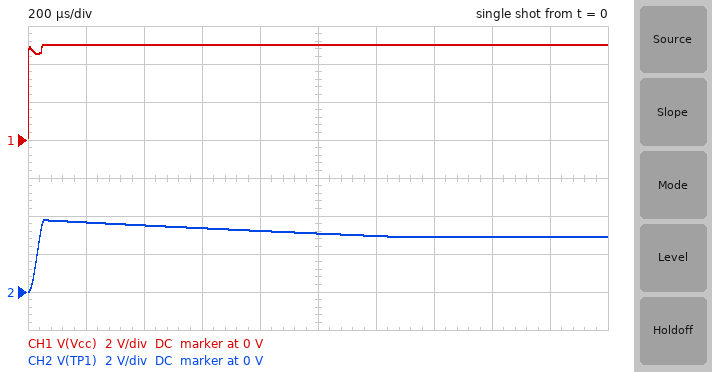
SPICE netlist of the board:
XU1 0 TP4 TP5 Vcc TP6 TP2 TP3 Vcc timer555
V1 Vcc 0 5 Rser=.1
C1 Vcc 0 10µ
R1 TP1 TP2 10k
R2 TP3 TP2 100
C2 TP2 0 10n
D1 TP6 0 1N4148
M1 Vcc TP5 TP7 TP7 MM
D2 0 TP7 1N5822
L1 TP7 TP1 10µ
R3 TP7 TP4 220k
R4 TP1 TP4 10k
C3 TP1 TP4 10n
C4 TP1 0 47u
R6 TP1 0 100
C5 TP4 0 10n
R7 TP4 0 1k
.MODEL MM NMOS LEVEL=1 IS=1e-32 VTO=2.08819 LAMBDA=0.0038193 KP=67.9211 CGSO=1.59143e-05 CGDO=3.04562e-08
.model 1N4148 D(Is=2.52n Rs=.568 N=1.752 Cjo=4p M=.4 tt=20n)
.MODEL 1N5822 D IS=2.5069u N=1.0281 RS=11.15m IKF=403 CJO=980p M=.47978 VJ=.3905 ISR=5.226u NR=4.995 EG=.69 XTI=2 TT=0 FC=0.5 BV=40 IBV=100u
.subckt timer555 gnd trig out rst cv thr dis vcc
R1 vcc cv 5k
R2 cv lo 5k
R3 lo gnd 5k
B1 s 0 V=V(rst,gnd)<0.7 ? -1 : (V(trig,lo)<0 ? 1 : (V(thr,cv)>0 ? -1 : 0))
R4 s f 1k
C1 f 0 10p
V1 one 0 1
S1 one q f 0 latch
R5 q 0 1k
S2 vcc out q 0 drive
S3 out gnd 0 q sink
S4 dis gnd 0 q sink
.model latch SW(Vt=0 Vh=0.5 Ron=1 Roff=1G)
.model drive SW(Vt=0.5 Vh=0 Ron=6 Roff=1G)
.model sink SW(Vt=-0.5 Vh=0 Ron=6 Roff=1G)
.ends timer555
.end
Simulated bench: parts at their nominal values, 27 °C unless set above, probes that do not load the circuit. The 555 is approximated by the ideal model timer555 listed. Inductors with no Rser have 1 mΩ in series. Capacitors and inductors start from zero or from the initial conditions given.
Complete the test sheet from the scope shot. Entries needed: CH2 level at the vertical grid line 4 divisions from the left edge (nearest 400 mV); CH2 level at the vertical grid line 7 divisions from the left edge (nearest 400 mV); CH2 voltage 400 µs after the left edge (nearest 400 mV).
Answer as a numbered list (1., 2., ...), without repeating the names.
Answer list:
1. 3.2 V
2. 2.8 V
3. 3.6 V
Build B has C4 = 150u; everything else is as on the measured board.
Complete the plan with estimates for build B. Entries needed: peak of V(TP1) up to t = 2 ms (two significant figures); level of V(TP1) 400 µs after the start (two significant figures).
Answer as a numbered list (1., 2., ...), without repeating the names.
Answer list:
1. 3.0 V
2. 2.9 V
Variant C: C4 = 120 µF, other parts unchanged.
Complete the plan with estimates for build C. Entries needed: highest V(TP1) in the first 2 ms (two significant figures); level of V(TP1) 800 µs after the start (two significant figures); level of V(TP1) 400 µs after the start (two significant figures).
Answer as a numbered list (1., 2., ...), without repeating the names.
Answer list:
1. 3.1 V
2. 2.9 V
3. 3.0 V
